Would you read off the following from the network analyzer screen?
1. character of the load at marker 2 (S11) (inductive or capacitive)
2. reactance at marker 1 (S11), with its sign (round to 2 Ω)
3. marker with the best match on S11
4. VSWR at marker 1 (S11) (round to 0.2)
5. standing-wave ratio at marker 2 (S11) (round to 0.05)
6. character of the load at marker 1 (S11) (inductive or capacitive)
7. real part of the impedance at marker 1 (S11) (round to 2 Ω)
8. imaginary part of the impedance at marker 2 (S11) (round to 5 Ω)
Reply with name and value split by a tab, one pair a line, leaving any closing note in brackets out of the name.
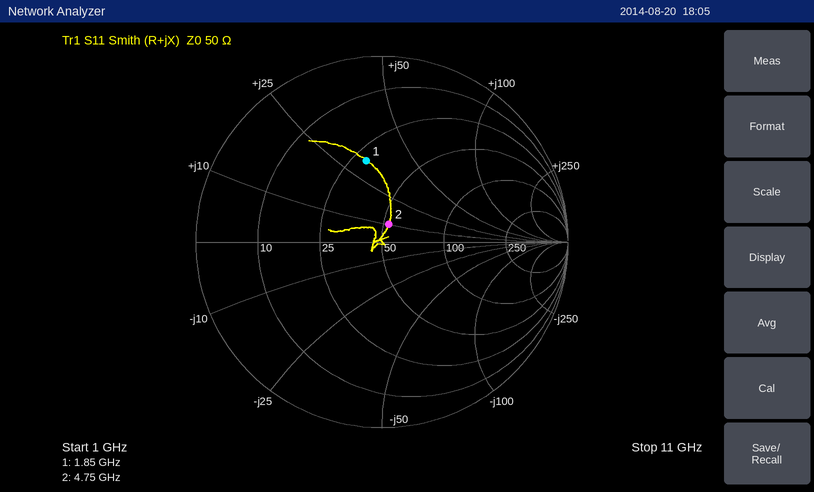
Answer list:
character of the load at marker 2 (S11)	inductive
reactance at marker 1 (S11), with its sign	+32 Ω
marker with the best match on S11	marker 2
VSWR at marker 1 (S11)	2.6
standing-wave ratio at marker 2 (S11)	1.25
character of the load at marker 1 (S11)	inductive
real part of the impedance at marker 1 (S11)	30 Ω
imaginary part of the impedance at marker 2 (S11)	+10 Ω
